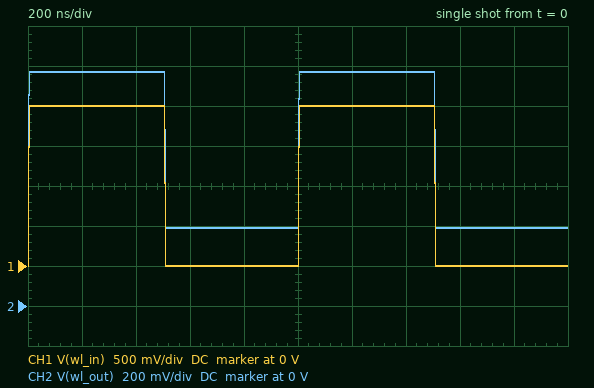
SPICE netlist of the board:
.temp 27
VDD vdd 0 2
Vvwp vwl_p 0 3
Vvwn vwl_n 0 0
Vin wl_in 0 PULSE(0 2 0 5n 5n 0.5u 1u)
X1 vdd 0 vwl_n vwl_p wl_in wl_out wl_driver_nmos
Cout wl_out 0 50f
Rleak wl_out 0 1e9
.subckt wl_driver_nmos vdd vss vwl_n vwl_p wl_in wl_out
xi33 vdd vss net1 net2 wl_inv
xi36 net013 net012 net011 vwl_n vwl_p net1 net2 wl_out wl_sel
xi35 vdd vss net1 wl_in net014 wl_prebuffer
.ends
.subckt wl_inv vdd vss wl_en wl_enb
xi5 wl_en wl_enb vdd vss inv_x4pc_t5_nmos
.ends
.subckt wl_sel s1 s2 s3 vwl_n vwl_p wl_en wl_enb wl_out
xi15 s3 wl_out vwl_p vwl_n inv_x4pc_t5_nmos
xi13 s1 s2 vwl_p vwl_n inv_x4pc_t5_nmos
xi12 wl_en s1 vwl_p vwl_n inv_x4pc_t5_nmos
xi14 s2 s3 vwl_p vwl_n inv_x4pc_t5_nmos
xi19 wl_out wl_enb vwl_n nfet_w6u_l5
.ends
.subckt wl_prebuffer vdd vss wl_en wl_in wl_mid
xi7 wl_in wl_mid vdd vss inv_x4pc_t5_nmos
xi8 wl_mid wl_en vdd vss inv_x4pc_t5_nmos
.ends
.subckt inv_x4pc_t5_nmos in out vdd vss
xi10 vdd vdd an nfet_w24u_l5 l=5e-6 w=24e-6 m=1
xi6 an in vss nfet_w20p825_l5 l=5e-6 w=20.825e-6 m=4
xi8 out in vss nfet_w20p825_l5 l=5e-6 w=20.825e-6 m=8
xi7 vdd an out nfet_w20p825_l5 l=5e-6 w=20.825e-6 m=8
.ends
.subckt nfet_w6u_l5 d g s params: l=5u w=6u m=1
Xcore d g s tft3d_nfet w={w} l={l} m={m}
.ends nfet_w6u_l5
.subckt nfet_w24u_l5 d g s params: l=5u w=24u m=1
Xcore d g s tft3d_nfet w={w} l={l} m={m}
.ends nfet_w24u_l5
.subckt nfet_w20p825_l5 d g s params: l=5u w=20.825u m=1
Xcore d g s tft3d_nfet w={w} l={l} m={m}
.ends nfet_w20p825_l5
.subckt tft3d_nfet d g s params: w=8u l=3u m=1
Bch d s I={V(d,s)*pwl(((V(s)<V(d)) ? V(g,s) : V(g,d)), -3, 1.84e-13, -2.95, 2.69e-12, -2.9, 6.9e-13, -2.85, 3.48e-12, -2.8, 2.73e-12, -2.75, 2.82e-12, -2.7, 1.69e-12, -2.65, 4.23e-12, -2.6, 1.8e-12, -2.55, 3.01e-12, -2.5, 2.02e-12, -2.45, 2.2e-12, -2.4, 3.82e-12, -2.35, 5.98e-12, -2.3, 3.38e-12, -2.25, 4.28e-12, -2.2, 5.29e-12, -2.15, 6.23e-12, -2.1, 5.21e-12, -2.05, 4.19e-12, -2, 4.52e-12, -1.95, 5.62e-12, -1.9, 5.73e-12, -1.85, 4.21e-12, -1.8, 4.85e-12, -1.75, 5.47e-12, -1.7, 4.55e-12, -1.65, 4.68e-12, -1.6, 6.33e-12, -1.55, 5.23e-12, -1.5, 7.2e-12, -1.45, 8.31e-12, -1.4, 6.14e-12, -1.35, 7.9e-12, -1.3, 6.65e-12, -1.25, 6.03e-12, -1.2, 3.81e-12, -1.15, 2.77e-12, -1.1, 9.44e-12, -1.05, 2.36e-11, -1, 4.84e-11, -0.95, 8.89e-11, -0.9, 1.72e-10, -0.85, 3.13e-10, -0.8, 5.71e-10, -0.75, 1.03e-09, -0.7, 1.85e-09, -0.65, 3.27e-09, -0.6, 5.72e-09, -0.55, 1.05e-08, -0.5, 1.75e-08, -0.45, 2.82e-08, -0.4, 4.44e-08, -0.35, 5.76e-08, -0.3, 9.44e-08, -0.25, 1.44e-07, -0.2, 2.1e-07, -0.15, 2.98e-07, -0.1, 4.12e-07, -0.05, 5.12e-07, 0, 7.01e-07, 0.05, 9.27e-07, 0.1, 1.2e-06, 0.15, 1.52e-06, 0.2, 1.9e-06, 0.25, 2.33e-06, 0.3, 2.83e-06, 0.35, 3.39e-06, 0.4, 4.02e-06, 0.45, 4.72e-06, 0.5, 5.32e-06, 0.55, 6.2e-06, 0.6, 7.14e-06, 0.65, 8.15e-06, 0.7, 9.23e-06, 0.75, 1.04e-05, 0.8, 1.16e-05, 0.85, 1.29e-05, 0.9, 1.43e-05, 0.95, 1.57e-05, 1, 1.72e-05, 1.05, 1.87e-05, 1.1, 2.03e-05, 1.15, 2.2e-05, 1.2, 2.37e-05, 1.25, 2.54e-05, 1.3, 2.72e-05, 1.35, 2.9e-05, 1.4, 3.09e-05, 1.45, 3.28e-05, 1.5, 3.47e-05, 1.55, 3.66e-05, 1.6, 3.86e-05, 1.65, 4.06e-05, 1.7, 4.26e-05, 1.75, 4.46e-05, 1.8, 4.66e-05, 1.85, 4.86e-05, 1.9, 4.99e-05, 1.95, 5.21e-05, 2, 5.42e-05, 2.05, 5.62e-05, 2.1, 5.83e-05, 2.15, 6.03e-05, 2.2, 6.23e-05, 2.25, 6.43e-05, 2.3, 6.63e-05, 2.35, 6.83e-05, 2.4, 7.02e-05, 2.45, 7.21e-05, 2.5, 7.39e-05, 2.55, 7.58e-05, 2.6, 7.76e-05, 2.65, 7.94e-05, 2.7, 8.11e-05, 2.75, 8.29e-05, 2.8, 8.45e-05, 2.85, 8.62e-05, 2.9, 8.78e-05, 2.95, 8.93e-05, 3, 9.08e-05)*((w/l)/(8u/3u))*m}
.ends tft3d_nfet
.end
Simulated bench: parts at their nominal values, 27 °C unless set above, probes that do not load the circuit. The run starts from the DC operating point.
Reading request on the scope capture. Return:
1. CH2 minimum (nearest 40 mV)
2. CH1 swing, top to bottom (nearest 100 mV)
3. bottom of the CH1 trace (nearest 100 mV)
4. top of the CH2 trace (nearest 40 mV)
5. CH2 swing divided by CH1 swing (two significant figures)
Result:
400 mV
2.0 V
0 V
1.16 V
0.39
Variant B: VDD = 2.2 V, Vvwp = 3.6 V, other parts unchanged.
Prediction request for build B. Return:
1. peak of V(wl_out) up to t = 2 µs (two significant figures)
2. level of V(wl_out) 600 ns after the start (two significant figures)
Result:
1.3 V
430 mV
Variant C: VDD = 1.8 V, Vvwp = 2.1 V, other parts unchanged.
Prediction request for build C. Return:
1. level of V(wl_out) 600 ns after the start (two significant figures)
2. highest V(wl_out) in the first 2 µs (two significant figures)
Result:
370 mV
850 mV
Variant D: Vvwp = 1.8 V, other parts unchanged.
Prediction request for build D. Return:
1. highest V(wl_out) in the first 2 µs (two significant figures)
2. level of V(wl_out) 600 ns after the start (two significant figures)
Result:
770 mV
360 mV
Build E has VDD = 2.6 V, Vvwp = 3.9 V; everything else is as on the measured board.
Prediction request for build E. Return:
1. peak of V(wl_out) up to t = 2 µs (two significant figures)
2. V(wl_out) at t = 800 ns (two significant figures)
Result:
1.5 V
450 mV
